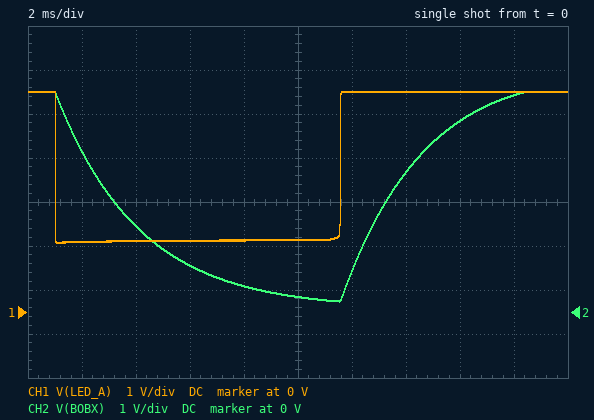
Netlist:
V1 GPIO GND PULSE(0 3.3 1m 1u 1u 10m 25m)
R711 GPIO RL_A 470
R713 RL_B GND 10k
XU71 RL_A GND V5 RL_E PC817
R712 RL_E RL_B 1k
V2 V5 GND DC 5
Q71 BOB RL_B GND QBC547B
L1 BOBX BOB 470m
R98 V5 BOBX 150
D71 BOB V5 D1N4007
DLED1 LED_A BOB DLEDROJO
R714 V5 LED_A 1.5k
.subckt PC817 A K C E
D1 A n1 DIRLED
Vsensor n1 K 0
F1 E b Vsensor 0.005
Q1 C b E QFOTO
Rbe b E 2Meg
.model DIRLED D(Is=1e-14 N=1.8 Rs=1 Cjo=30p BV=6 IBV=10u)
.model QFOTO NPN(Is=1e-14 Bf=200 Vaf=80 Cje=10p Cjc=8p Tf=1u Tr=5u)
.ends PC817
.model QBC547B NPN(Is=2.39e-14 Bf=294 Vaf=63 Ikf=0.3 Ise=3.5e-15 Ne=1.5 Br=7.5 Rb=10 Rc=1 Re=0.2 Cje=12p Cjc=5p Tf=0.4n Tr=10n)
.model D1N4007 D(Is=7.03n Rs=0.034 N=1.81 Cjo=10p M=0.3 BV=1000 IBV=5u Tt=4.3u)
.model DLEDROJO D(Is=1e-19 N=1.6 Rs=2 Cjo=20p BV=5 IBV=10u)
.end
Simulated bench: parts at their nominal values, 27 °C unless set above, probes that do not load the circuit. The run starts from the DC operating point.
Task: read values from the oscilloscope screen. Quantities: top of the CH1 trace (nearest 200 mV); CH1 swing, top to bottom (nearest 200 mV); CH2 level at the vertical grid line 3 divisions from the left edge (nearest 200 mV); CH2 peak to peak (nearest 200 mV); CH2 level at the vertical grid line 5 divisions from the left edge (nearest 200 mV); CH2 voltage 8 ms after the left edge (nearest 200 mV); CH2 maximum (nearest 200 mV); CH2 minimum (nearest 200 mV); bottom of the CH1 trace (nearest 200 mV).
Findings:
5.0 V
3.4 V
1.0 V
4.8 V
400 mV
600 mV
5.0 V
200 mV
1.6 V
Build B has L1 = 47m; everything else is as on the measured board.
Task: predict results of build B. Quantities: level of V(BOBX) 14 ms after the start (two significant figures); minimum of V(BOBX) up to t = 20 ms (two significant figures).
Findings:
5.0 V
69 mV
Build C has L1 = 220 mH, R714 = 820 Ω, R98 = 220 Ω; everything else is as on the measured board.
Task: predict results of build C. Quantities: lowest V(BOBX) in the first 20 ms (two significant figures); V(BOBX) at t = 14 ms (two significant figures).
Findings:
54 mV
5.0 V
